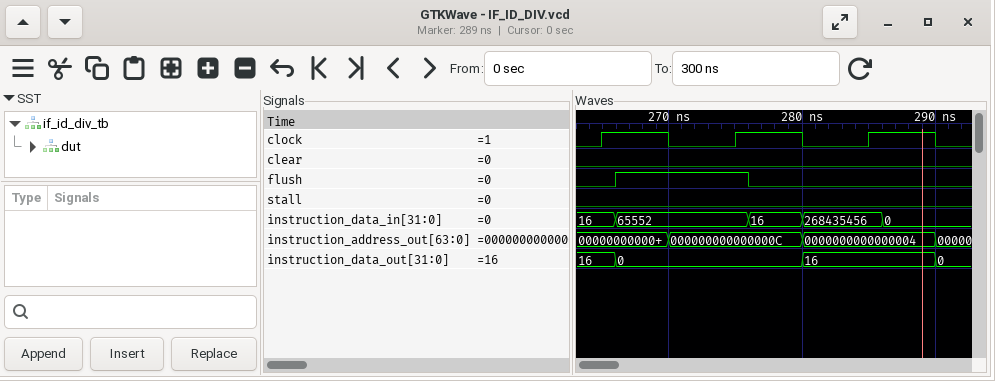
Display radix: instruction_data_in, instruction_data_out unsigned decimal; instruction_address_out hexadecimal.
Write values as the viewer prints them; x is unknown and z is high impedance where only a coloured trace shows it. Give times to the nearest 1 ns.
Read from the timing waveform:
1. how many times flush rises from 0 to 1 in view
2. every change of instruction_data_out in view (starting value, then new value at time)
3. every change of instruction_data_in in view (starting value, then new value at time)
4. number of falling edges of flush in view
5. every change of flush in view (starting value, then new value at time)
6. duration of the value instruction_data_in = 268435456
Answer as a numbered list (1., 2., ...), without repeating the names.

1. 1
2. 16, 0 at 266 ns, 16 at 280 ns, 0 at 290 ns
3. 16, 65552 at 266 ns, 16 at 276 ns, 268435456 at 280 ns, 0 at 286 ns
4. 1
5. 0, 1 at 266 ns, 0 at 276 ns
6. 6 ns
